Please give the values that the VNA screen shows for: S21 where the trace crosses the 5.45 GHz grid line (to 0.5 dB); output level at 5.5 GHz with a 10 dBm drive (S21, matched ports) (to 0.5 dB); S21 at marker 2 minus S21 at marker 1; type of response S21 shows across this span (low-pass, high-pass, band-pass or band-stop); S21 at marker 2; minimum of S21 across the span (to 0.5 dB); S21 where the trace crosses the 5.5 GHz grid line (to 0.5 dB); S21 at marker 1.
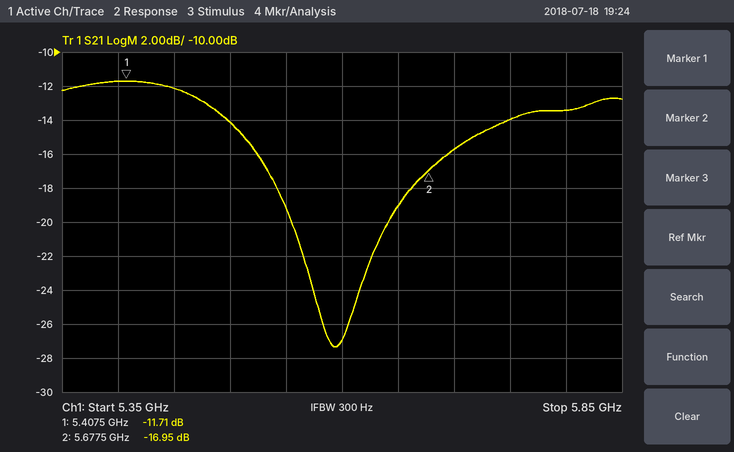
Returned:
-12.0 dB
-4.0 dBm
-5.24 dB
band-stop
-16.95 dB
-27.5 dB
-14.0 dB
-11.71 dB
